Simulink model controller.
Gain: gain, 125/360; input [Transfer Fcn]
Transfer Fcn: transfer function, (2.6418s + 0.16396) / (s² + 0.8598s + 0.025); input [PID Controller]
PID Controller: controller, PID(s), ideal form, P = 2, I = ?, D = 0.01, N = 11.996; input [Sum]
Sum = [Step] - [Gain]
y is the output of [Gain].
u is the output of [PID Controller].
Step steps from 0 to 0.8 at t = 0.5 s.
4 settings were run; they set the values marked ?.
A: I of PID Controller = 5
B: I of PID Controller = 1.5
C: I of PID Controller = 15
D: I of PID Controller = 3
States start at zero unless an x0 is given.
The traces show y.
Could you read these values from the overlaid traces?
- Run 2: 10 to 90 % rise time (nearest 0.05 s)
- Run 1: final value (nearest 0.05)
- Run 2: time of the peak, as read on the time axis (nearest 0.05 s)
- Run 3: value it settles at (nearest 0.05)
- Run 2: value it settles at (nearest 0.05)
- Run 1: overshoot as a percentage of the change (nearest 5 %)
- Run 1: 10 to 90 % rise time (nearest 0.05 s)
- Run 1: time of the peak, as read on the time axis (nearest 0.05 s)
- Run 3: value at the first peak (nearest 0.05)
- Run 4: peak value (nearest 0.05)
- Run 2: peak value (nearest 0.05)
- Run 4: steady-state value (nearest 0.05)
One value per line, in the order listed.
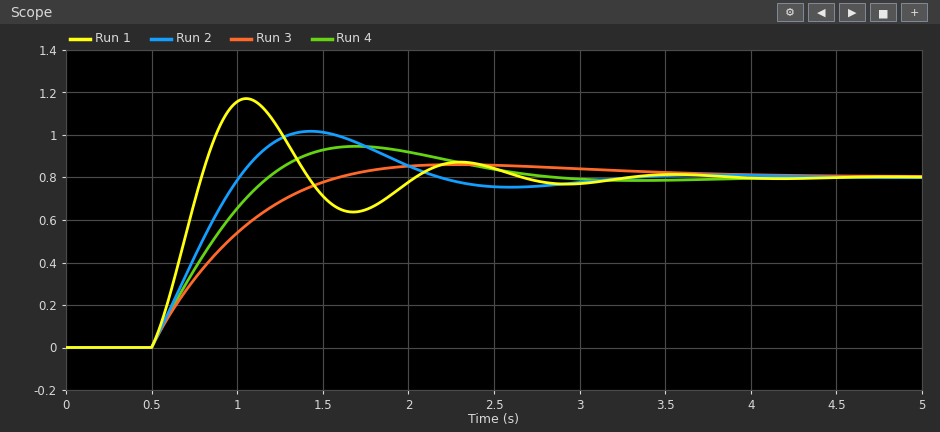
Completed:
0.40 s
0.80
1.45 s
0.80
0.80
45 %
0.20 s
1.05 s
0.85
0.95
1.00
0.80
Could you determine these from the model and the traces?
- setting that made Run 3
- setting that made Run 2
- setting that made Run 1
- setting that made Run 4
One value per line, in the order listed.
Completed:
B
A
C
D
